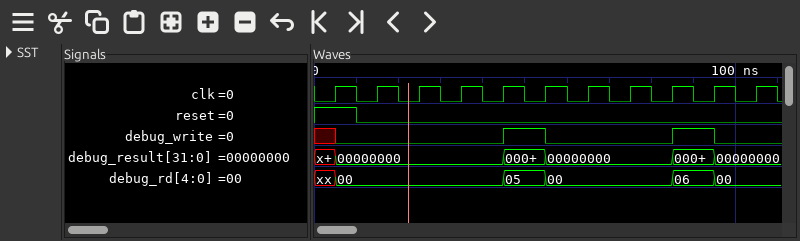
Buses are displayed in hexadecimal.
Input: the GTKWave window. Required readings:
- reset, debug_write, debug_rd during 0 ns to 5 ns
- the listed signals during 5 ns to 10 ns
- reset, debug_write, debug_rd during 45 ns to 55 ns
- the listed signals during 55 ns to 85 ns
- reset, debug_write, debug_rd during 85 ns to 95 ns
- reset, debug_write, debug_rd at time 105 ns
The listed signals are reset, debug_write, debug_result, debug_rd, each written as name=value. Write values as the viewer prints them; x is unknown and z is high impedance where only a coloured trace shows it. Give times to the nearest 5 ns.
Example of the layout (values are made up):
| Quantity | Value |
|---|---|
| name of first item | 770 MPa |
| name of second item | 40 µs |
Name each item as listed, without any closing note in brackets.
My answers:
| Quantity | Value |
|---|---|
| reset, debug_write, debug_rd during 0 ns to 5 ns | reset=1, debug_write=x, debug_rd=xx |
| the listed signals during 5 ns to 10 ns | reset=1, debug_write=0, debug_result=00000000, debug_rd=00 |
| reset, debug_write, debug_rd during 45 ns to 55 ns | reset=0, debug_write=1, debug_rd=05 |
| the listed signals during 55 ns to 85 ns | reset=0, debug_write=0, debug_result=00000000, debug_rd=00 |
| reset, debug_write, debug_rd during 85 ns to 95 ns | reset=0, debug_write=1, debug_rd=06 |
| reset, debug_write, debug_rd at time 105 ns | reset=0, debug_write=0, debug_rd=00 |
